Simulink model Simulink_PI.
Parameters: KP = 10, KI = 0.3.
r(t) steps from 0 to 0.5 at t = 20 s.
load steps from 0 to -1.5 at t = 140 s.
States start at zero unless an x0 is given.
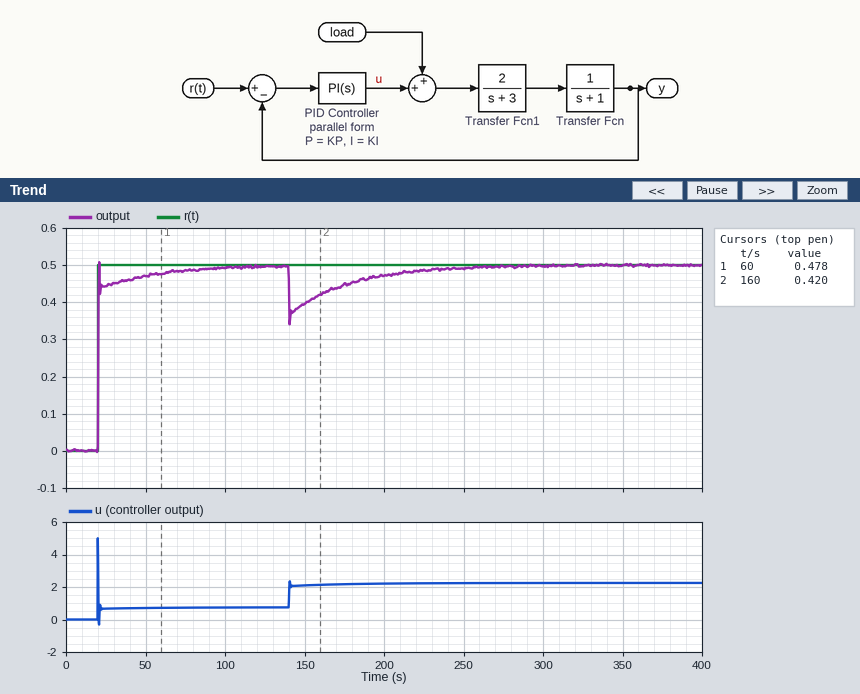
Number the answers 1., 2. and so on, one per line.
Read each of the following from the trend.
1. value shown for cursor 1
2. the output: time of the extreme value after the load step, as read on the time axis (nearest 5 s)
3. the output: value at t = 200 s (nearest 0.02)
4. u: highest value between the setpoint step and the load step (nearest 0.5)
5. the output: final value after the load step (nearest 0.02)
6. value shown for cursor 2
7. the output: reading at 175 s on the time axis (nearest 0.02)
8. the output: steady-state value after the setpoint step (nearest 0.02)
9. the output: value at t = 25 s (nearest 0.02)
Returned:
1. 0.478
2. 140 s
3. 0.48
4. 5.0
5. 0.50
6. 0.420
7. 0.44
8. 0.50
9. 0.44
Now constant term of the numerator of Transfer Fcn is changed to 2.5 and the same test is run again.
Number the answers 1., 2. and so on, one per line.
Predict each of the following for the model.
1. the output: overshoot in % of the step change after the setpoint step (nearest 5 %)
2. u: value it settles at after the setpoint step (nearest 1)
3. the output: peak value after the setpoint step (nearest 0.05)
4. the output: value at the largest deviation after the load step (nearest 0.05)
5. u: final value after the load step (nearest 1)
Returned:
1. 30 %
2. 0
3. 0.65
4. 0.30
5. 2
